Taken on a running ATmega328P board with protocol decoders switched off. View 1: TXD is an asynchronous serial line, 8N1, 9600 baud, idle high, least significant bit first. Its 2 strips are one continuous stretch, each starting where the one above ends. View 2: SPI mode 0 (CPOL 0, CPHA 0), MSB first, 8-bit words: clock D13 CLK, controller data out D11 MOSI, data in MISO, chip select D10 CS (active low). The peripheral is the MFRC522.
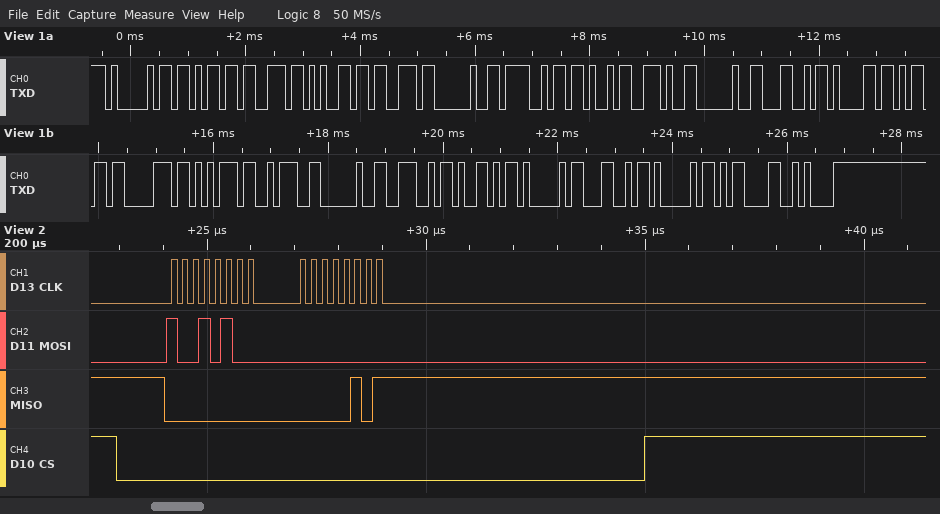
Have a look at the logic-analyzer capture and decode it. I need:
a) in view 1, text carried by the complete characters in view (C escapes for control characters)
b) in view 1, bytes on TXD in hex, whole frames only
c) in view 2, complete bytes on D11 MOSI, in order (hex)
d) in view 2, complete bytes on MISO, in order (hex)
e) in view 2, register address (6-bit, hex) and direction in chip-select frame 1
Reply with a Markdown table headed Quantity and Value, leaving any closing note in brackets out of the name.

| Quantity | Value |
|---|---|
| in view 1, text carried by the complete characters in view | "Akses OK. Lampu: NYALA\r\n" |
| in view 1, bytes on TXD in hex, whole frames only | 41 6B 73 65 73 20 4F 4B 2E 20 4C 61 6D 70 75 3A 20 4E 59 41 4C 41 0D 0A |
| in view 2, complete bytes on D11 MOSI, in order | 0x94 0x00 |
| in view 2, complete bytes on MISO, in order | 0x00 0x05 |
| in view 2, register address (6-bit, hex) and direction in chip-select frame 1 | 0x0A read |
